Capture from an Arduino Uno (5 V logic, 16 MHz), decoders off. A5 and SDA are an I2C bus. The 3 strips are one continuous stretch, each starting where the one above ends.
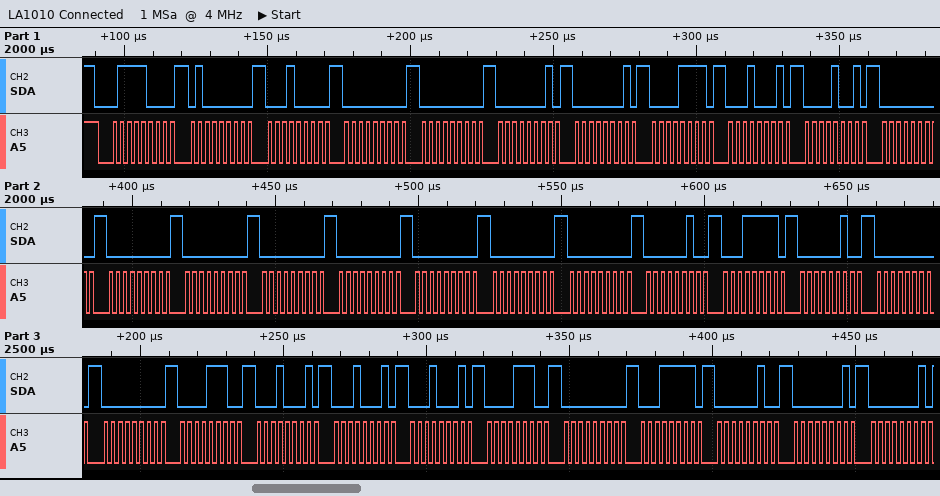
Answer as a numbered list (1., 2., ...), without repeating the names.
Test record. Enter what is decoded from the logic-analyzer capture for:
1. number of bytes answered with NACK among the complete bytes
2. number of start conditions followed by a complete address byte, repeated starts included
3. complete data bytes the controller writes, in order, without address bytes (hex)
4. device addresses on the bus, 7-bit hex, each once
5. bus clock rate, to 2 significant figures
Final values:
1. 0
2. 1
3. 40 10 00 00 01 01 0F 11 09 00 00 00 00 00 00 00 00 02 1F 02 00 00 0E 11 11 11 0E 00 1F 02 01 01
4. 0x3C
5. 400 kHz
